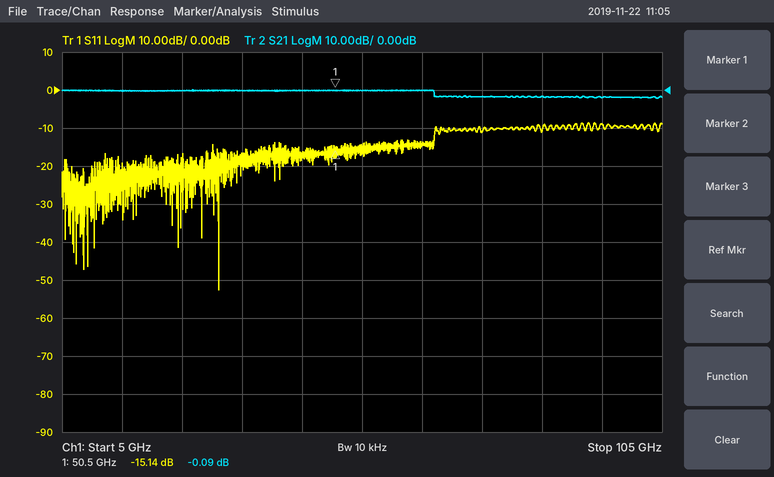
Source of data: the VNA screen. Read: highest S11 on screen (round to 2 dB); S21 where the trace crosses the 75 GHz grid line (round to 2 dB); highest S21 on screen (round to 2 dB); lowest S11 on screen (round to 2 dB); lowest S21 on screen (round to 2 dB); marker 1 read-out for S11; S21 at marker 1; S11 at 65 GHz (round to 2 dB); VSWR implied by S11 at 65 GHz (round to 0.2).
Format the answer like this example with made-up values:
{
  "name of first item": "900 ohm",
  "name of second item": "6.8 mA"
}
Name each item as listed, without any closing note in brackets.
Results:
{
  "highest S11 on screen": "-8 dB",
  "S21 where the trace crosses the 75 GHz grid line": "-2 dB",
  "highest S21 on screen": "0 dB",
  "lowest S11 on screen": "-52 dB",
  "lowest S21 on screen": "-2 dB",
  "marker 1 read-out for S11": "-15.14 dB",
  "S21 at marker 1": "-0.09 dB",
  "S11 at 65 GHz": "-14 dB",
  "VSWR implied by S11 at 65 GHz": "1.4"
}
